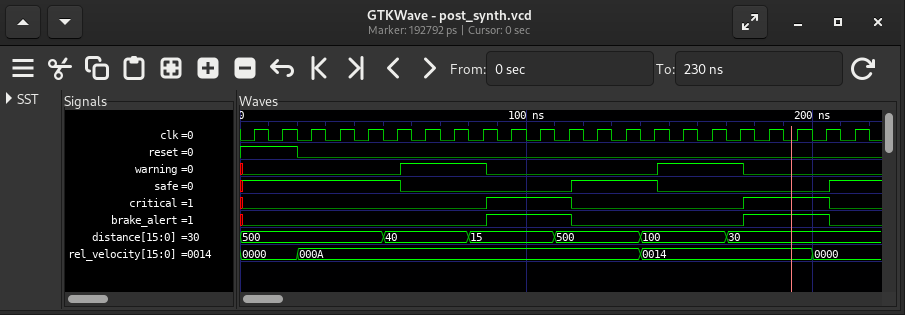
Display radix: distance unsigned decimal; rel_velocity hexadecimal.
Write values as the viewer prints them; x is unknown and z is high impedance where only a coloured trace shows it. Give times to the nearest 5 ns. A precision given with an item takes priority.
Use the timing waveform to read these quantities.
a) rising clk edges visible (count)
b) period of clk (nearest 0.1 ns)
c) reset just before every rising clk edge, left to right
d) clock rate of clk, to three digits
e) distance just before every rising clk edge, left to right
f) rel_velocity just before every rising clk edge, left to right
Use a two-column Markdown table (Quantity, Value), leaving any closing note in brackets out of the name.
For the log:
| Quantity | Value |
|---|---|
| rising clk edges visible | 22 |
| period of clk | 10 ns |
| reset just before every rising clk edge, left to right | 1 1 0 0 0 0 0 0 0 0 0 0 0 0 0 0 0 0 0 0 0 0 |
| clock rate of clk, to three digits | 100 MHz |
| distance just before every rising clk edge, left to right | 500, 500, 500, 500, 500, 40, 40, 40, 15, 15, 15, 500, 500, 500, 100, 100, 100, 30, 30, 30, 30, 30 |
| rel_velocity just before every rising clk edge, left to right | 0000, 0000, 000A, 000A, 000A, 000A, 000A, 000A, 000A, 000A, 000A, 000A, 000A, 000A, 0014, 0014, 0014, 0014, 0014, 0014, 0000, 0000 |
